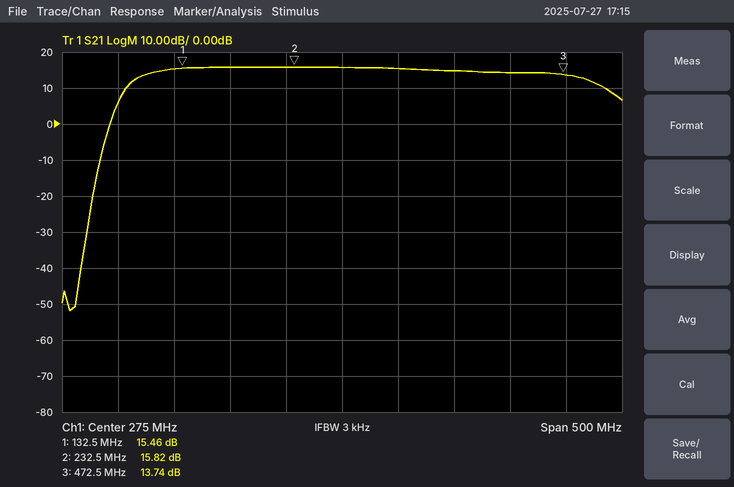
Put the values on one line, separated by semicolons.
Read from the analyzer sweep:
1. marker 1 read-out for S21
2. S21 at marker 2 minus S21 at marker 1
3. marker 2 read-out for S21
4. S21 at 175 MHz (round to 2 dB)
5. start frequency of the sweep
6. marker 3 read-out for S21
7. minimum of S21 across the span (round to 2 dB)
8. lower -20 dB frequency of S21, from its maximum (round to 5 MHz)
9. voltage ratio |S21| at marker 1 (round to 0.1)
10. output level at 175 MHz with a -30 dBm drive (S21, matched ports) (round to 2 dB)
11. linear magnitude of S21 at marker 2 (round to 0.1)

15.46 dB; 0.36 dB; 15.82 dB; 16 dB; 25 MHz; 13.74 dB; -52 dB; 65 MHz; 5.9; -14 dBm; 6.2
